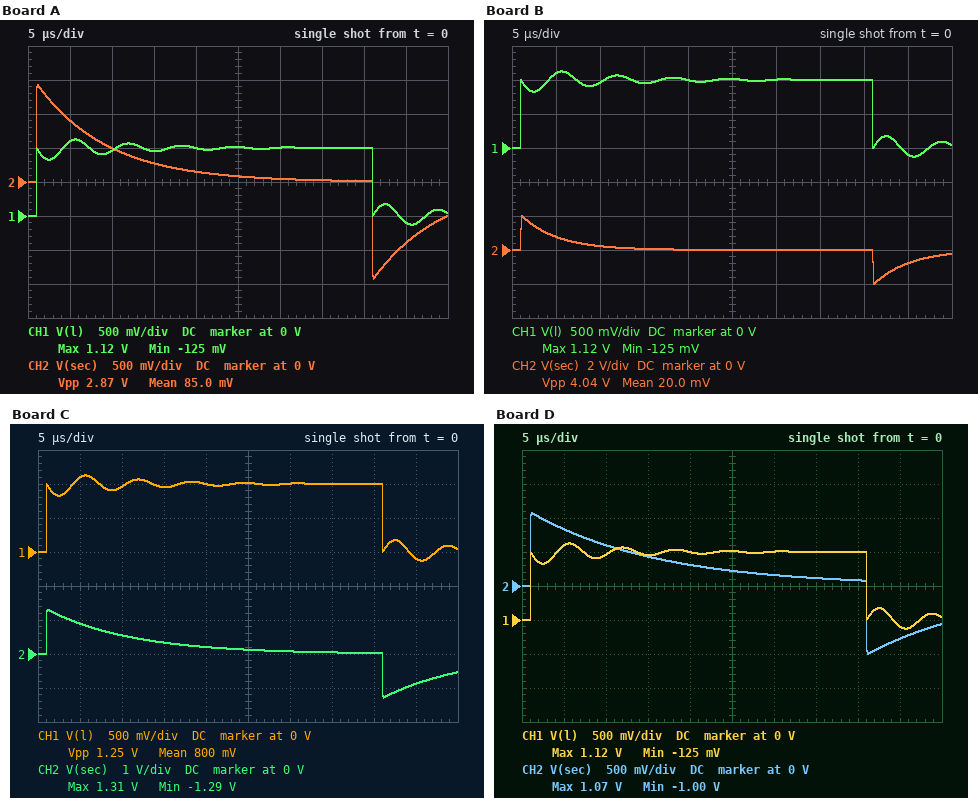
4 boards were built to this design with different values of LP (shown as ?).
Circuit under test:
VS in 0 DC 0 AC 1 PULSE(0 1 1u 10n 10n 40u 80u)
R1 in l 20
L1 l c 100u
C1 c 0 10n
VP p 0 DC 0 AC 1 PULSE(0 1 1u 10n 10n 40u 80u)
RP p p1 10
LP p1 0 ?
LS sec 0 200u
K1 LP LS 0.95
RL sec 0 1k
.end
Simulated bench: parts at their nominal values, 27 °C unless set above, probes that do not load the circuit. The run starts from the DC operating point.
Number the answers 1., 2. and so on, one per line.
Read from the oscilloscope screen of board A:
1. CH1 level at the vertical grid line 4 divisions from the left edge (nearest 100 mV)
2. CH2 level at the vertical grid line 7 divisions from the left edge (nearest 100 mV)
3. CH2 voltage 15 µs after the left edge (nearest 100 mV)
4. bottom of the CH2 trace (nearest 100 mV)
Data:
1. 1.0 V
2. 0 V
3. 300 mV
4. -1.4 V
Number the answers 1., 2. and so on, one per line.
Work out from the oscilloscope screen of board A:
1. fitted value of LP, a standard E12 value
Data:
1. 82 µH
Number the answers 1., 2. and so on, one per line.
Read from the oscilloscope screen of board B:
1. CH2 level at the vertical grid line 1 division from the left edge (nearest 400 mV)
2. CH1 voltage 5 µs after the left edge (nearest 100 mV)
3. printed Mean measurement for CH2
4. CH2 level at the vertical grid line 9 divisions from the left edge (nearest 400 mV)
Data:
1. 800 mV
2. 1.1 V
3. 20.0 mV
4. -800 mV
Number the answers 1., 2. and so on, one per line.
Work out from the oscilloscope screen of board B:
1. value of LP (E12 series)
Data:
1. 39 µH
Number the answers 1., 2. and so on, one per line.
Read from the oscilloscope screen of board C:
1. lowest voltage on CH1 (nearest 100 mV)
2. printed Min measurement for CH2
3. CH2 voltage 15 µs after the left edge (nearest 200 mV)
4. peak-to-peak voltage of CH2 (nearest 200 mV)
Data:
1. -100 mV
2. -1.29 V
3. 400 mV
4. 2.6 V
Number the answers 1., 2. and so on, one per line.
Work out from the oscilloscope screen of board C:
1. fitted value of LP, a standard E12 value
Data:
1. 100 µH
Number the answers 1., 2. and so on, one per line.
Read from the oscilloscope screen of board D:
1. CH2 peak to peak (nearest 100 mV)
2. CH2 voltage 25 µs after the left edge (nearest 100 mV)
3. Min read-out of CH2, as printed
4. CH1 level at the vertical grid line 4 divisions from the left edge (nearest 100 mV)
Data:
1. 2.1 V
2. 200 mV
3. -1.00 V
4. 1.0 V
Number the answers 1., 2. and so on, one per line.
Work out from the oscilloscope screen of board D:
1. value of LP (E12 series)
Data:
1. 150 µH
